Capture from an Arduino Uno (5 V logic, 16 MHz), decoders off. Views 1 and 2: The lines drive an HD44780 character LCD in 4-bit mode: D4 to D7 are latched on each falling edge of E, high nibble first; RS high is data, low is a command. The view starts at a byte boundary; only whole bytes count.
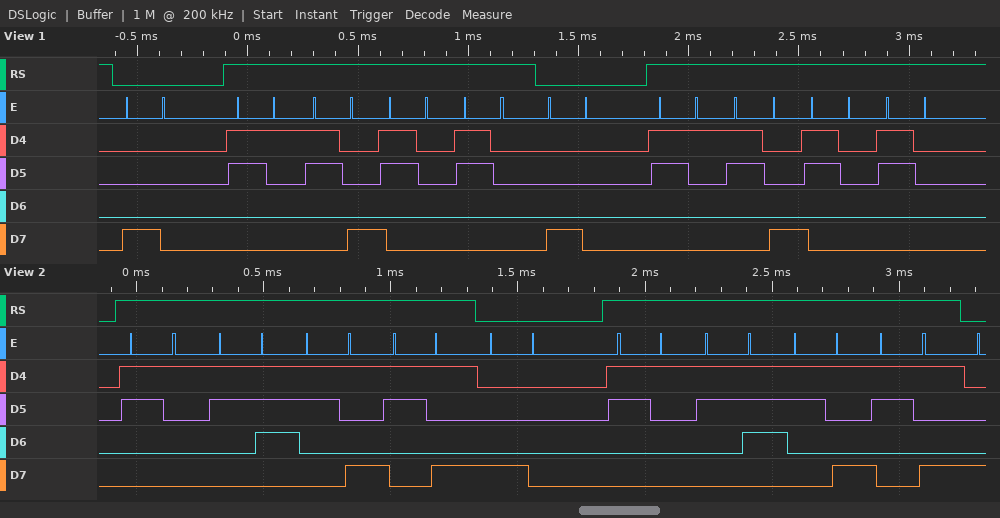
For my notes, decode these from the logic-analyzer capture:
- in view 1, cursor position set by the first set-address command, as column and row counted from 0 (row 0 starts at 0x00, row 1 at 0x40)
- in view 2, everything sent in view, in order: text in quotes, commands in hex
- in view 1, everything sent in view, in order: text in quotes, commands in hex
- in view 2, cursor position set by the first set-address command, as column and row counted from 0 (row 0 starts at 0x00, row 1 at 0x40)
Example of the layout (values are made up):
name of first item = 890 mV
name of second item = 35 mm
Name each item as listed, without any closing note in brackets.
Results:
in view 1, cursor position set by the first set-address command, as column and row counted from 0 = column 0, row 0
in view 2, everything sent in view, in order: text in quotes, commands in hex = "1799" 0x80 "1799"
in view 1, everything sent in view, in order: text in quotes, commands in hex = 0x80 "1800" 0x80 "1800"
in view 2, cursor position set by the first set-address command, as column and row counted from 0 = column 0, row 0
